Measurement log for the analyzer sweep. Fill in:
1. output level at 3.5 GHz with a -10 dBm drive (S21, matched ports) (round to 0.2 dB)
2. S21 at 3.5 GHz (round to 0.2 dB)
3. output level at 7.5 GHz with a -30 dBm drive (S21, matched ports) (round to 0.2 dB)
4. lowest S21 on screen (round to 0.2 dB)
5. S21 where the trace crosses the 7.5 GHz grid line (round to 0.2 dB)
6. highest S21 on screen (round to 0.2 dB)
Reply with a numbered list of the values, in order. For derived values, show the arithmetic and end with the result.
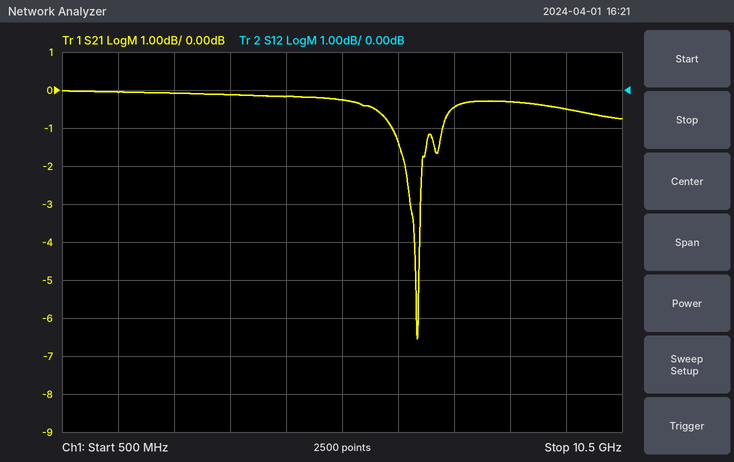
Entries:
1. -10 dBm + (-0.2 dB) = -10.2 dBm
2. -0.2 dB
3. -30 dBm + (-0.4 dB) = -30.4 dBm
4. -6.6 dB
5. -0.4 dB
6. 0.0 dB
